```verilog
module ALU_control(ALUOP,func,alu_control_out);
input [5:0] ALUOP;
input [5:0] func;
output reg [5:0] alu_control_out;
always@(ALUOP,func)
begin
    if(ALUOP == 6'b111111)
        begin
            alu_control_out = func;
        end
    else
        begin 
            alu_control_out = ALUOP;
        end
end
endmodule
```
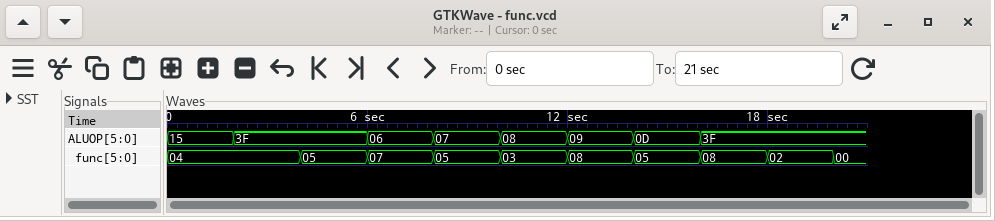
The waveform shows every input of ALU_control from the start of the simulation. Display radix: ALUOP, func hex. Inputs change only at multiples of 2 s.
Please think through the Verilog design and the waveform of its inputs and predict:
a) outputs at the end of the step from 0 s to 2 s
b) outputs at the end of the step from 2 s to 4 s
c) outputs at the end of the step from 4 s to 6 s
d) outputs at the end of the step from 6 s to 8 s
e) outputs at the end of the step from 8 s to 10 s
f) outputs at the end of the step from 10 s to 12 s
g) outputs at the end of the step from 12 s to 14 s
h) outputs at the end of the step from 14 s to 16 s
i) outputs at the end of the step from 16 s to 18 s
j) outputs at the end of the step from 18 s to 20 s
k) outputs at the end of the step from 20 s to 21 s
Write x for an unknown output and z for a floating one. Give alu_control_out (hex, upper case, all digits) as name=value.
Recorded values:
alu_control_out=15
alu_control_out=04
alu_control_out=05
alu_control_out=06
alu_control_out=07
alu_control_out=08
alu_control_out=09
alu_control_out=0D
alu_control_out=08
alu_control_out=02
alu_control_out=00
